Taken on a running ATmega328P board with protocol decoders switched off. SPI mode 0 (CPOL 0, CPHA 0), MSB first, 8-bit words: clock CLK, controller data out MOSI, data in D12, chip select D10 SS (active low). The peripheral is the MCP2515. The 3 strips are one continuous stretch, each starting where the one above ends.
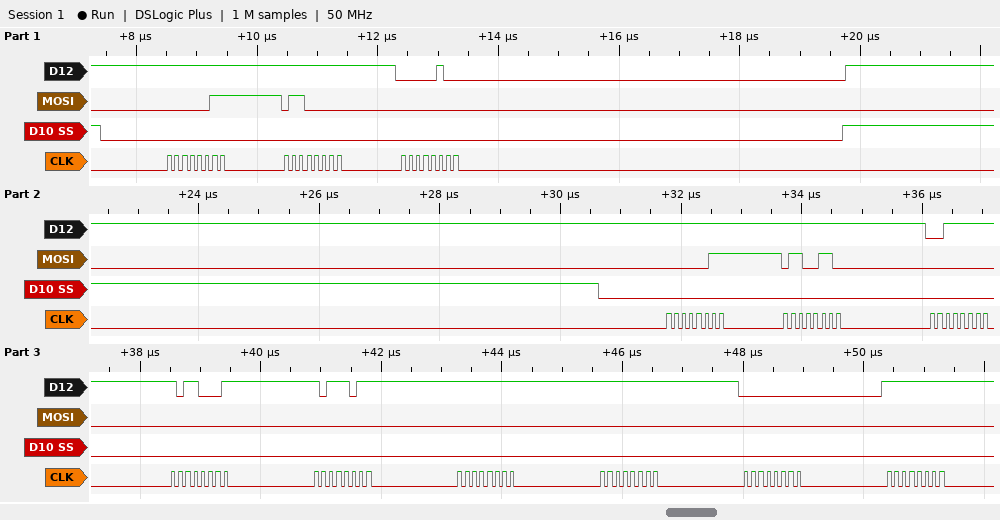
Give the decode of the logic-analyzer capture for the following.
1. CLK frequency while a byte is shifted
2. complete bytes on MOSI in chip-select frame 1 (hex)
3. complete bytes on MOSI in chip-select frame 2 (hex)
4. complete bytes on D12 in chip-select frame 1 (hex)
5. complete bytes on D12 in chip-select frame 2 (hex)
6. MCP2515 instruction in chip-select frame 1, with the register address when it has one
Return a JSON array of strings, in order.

["8 MHz", "03 60 00", "03 66 00 00 00 00 00 00 00", "FF FF 04", "FF FF 3F B1 BB FF FF 00 FF", "READ 0x60"]
